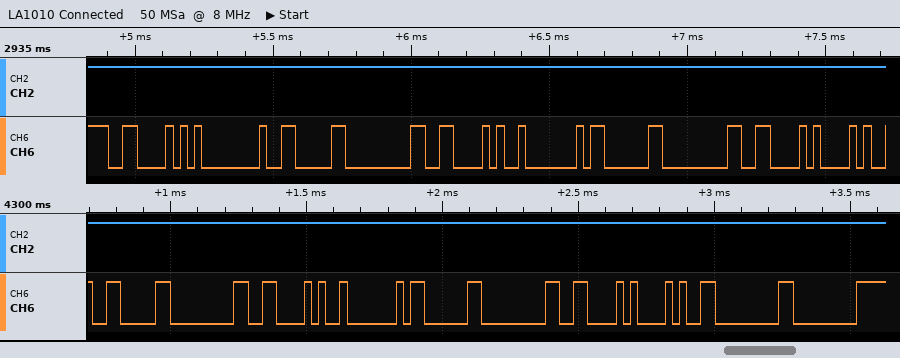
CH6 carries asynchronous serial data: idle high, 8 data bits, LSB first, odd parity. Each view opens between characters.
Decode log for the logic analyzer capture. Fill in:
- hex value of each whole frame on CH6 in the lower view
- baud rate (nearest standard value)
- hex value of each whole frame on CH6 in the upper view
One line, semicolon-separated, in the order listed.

06, 00, 86, 02, 03, 00, 86, 28, 00, 00; 38400 baud; 86, 01, 06, 00, 86, 02, 03, 00, 86
